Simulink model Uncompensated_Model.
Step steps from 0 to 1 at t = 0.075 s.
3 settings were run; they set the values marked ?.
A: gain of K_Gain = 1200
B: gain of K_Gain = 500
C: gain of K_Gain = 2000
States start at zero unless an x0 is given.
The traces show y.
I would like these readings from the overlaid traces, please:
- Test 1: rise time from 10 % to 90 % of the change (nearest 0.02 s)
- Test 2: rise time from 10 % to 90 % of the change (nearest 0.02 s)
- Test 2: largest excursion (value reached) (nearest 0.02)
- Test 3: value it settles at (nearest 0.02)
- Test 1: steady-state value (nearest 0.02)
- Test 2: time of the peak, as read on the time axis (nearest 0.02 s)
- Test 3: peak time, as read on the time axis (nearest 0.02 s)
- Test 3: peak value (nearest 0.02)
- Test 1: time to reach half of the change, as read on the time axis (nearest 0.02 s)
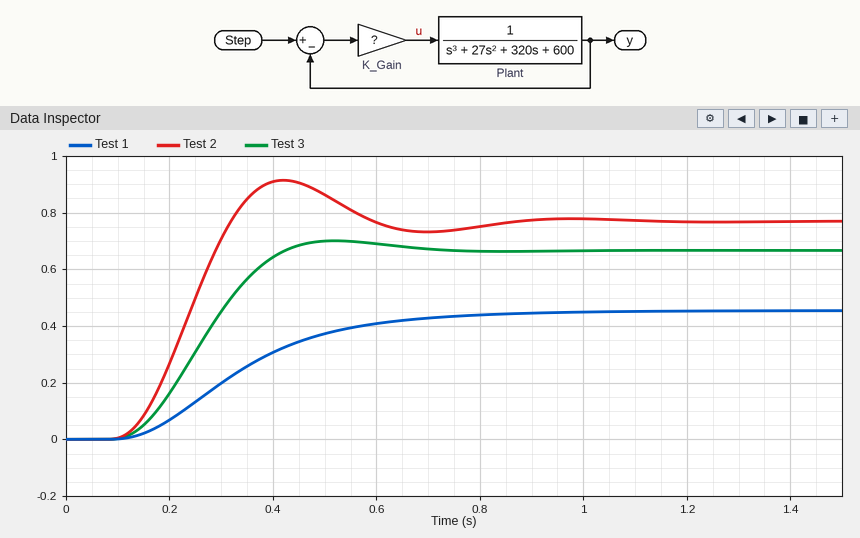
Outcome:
0.42 s
0.14 s
0.92
0.66
0.46
0.42 s
0.52 s
0.70
0.32 s
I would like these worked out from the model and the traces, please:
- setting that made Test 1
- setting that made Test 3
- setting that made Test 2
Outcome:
B
A
C
